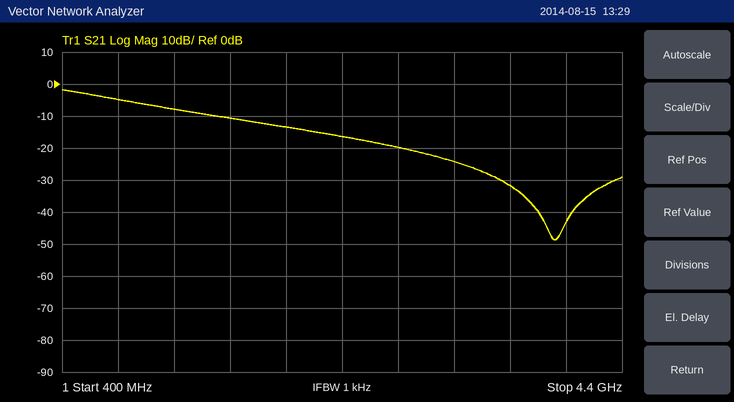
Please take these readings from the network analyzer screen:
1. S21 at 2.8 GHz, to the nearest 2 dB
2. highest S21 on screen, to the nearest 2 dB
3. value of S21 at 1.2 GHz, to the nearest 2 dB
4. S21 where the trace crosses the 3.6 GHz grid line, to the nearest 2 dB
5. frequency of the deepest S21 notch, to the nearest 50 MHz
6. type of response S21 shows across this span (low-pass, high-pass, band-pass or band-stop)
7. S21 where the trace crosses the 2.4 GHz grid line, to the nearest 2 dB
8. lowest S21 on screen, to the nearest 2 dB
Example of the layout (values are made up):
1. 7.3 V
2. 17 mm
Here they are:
1. -20 dB
2. -2 dB
3. -8 dB
4. -32 dB
5. 3.90 GHz
6. low-pass
7. -16 dB
8. -48 dB
